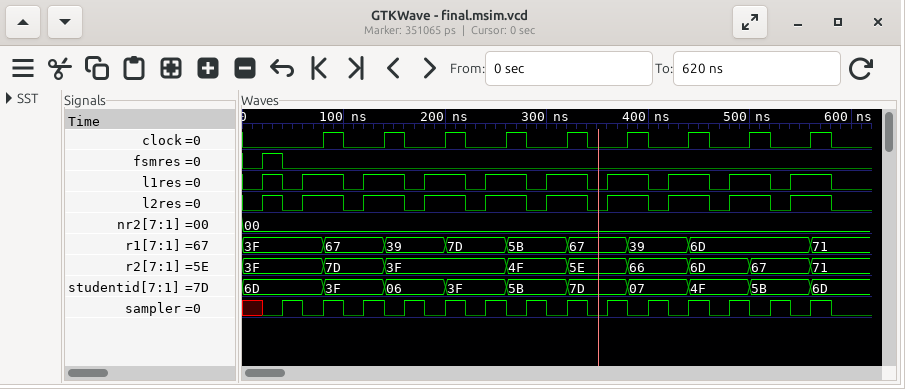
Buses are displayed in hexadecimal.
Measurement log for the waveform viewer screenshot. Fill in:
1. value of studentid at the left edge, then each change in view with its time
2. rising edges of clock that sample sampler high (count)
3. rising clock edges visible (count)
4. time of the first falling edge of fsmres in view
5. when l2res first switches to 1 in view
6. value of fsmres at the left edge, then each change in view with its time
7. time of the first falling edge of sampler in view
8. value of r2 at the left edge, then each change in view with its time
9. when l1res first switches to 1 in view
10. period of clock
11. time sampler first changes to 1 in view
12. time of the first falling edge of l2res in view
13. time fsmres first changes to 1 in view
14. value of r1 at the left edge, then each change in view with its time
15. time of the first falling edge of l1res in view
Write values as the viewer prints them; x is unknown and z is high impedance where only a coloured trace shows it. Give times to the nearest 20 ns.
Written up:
6D, 3F at 80 ns, 06 at 140 ns, 3F at 200 ns, 5B at 260 ns, 7D at 320 ns, 07 at 380 ns, 4F at 440 ns, 5B at 500 ns, 6D at 560 ns
4
9
40 ns
20 ns
0, 1 at 20 ns, 0 at 40 ns
60 ns
3F, 7D at 80 ns, 3F at 140 ns, 4F at 260 ns, 5E at 320 ns, 66 at 380 ns, 6D at 440 ns, 67 at 500 ns, 71 at 560 ns
20 ns
60 ns
40 ns
40 ns
20 ns
3F, 67 at 80 ns, 39 at 140 ns, 7D at 200 ns, 5B at 260 ns, 67 at 320 ns, 39 at 380 ns, 6D at 440 ns, 71 at 560 ns
40 ns
